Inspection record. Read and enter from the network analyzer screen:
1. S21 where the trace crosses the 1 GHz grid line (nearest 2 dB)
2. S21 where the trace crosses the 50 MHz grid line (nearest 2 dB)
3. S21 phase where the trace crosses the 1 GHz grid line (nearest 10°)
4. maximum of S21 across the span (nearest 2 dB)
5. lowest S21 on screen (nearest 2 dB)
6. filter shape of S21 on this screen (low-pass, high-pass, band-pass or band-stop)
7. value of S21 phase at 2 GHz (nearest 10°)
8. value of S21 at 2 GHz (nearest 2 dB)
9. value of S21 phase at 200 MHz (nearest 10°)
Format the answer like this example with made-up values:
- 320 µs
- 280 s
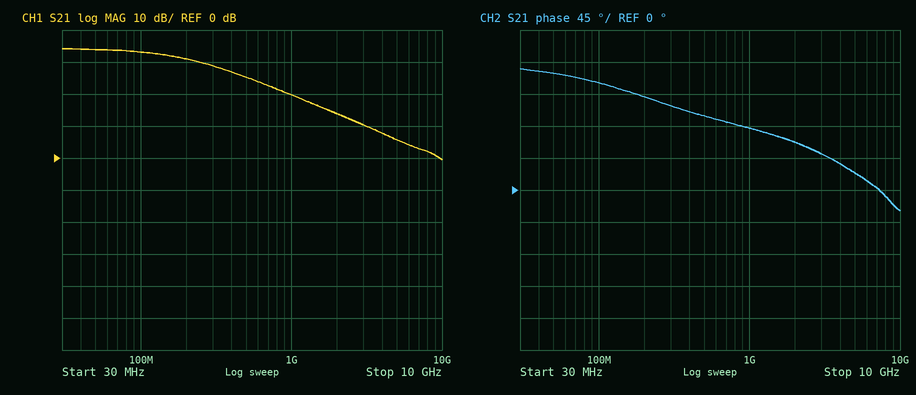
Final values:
- 20 dB
- 34 dB
- 90°
- 34 dB
- 0 dB
- low-pass
- 70°
- 14 dB
- 130°
